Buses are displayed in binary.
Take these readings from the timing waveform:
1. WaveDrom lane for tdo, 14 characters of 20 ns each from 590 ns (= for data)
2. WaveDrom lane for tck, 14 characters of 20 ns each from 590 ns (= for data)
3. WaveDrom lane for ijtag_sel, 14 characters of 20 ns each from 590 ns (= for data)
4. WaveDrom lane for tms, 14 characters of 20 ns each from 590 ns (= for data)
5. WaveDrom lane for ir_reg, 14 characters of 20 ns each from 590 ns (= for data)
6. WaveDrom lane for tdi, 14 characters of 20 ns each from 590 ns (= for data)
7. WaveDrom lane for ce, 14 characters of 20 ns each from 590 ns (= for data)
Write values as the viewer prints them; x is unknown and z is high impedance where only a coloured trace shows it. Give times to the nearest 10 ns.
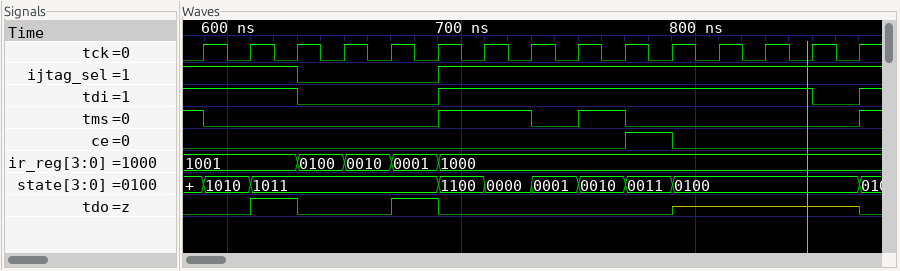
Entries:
{name: 'tdo', wave: '010.10....z...'}
{name: 'tck', wave: 'p.............'}
{name: 'ijtag_sel', wave: '1.0..1........'}
{name: 'tms', wave: '0....1.010....'}
{name: 'ir_reg', wave: '=.====........', data: '1001 0100 0010 0001 1000'}
{name: 'tdi', wave: '1.0..1.......0'}
{name: 'ce', wave: '0........10...'}
